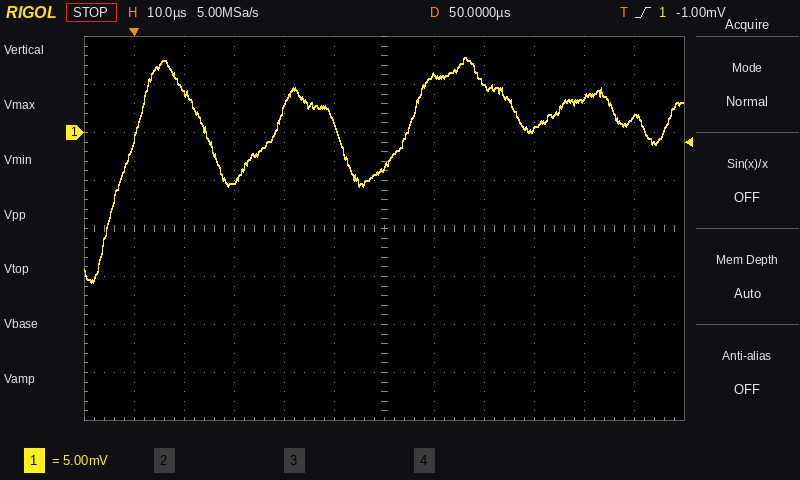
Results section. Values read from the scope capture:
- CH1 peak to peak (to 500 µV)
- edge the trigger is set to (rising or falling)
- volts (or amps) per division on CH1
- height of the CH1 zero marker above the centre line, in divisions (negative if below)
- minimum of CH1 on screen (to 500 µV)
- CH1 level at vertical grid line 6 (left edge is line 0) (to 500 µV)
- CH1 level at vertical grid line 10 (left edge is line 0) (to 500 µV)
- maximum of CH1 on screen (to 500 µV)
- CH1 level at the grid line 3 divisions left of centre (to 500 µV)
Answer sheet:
23.5 mV
rising
5 mV
+2.0 div
-15.5 mV
-3.5 mV
3.5 mV
8.0 mV
-5.0 mV
